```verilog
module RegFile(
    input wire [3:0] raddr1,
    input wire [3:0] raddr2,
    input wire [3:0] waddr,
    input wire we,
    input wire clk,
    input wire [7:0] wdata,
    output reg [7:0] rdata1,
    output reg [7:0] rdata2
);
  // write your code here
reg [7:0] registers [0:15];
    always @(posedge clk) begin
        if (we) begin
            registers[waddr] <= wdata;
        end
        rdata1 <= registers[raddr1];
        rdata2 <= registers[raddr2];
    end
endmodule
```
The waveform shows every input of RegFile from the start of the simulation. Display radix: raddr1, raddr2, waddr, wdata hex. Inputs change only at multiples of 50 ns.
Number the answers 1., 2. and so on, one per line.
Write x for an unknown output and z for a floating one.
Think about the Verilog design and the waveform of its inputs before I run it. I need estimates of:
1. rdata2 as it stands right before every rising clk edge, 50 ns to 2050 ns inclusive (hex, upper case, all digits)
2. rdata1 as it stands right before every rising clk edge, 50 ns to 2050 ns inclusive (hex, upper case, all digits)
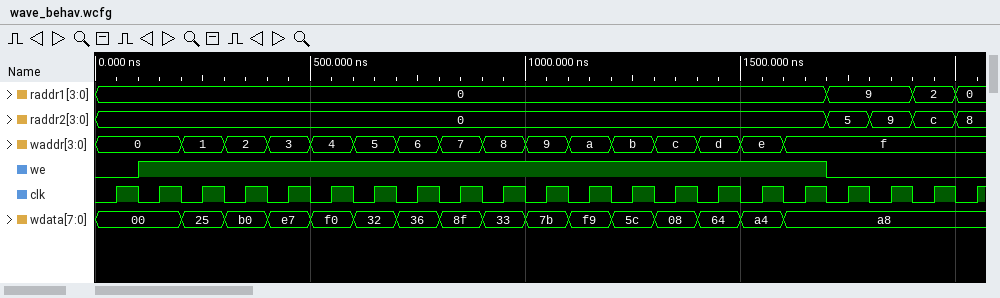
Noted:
1. x, x, x, 00, 00, 00, 00, 00, 00, 00, 00, 00, 00, 00, 00, 00, 00, 00, 32, 7B, 08
2. x, x, x, 00, 00, 00, 00, 00, 00, 00, 00, 00, 00, 00, 00, 00, 00, 00, 7B, 7B, B0
